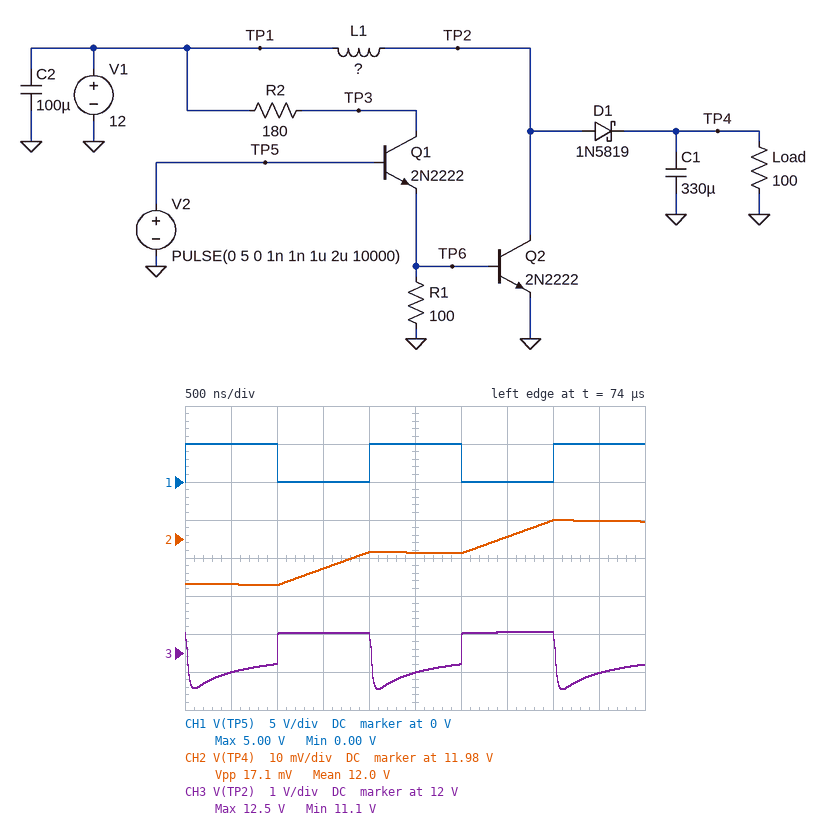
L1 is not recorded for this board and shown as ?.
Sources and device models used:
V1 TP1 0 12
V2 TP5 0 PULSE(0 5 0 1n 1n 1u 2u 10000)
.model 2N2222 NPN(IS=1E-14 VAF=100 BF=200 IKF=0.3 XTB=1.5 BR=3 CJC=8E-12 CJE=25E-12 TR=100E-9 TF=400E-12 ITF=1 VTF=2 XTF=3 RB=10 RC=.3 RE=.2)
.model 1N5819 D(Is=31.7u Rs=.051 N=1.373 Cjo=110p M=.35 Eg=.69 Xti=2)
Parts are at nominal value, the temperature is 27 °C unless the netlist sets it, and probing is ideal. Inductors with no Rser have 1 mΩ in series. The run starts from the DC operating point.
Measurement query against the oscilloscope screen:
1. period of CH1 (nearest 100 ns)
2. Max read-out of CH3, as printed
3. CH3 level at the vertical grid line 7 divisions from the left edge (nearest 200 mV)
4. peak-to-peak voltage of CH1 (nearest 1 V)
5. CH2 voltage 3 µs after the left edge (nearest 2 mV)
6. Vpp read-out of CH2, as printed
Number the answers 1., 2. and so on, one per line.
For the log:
1. 2.0 µs
2. 12.5 V
3. 12.6 V
4. 5 V
5. 11.976 V
6. 17.1 mV
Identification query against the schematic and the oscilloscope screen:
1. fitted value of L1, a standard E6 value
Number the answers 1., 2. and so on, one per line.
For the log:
1. 47 µH
